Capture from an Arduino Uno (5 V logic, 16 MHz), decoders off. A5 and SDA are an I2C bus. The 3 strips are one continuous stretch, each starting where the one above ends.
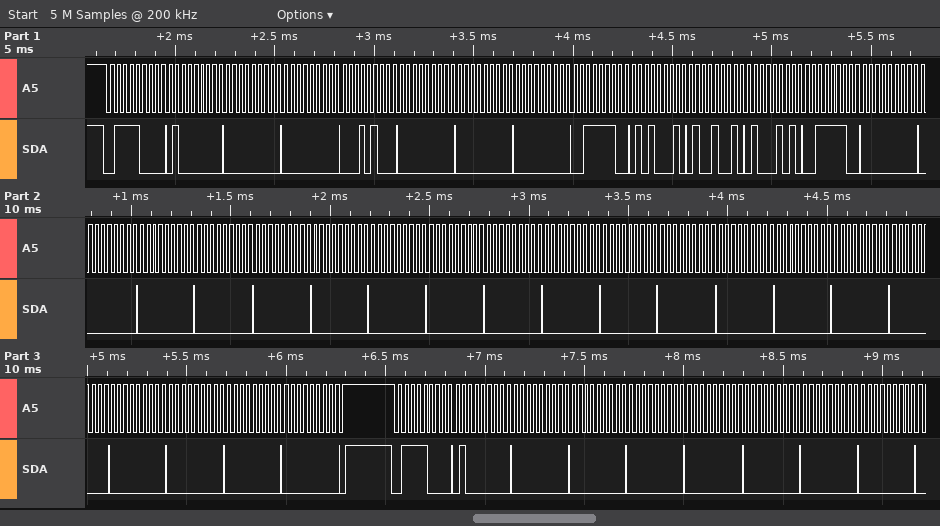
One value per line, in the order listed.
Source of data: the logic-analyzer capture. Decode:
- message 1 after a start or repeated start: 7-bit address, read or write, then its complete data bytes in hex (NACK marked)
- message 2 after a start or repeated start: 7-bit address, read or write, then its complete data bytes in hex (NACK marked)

0x3C write: 40 00 00 14 00 00 00 3E 51 49 45 3E 00 00 00 00 00 00 00 00 00 00 00 00 00 00 00 00 00 00 00 00
0x3C write: 40 00 00 00 00 00 00 00
